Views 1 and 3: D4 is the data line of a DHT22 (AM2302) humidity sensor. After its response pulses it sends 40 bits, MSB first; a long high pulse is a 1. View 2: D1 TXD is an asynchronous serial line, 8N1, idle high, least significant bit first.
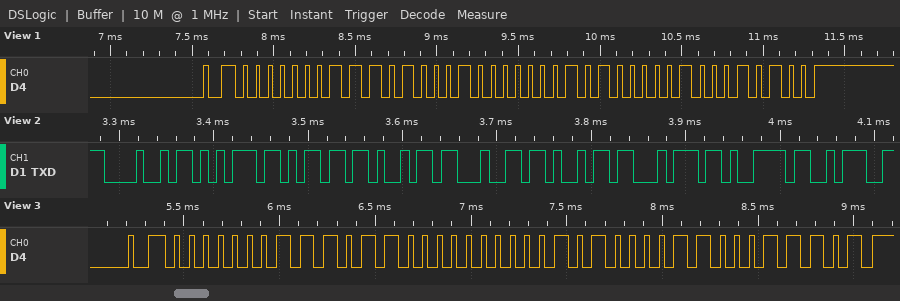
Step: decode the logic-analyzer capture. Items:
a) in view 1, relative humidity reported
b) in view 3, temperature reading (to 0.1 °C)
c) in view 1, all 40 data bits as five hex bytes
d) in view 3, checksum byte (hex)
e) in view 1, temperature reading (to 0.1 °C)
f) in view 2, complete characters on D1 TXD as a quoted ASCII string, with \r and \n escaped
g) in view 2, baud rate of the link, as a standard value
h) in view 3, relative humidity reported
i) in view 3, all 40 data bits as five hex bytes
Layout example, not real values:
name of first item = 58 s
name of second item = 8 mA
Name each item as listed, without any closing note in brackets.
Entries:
in view 1, relative humidity reported = 46.5 %
in view 3, temperature reading = 32.3 °C
in view 1, all 40 data bits as five hex bytes = 01 D1 01 41 14
in view 3, checksum byte = 0x1D
in view 1, temperature reading = 32.1 °C
in view 2, complete characters on D1 TXD as a quoted ASCII string, with \r and \n escaped = "Humidity:"
in view 2, baud rate of the link, as a standard value = 115200 baud
in view 3, relative humidity reported = 47.2 %
in view 3, all 40 data bits as five hex bytes = 01 D8 01 43 1D
